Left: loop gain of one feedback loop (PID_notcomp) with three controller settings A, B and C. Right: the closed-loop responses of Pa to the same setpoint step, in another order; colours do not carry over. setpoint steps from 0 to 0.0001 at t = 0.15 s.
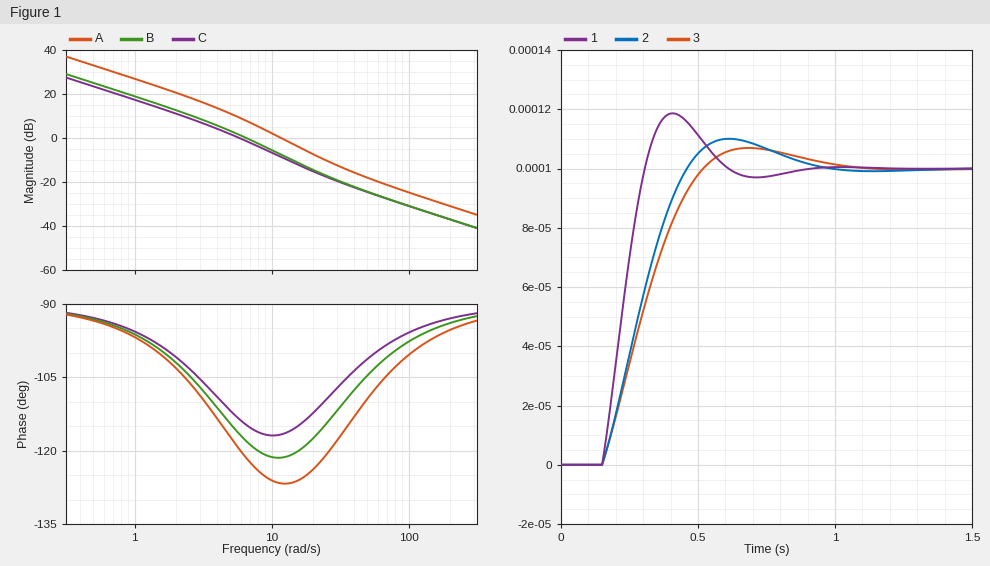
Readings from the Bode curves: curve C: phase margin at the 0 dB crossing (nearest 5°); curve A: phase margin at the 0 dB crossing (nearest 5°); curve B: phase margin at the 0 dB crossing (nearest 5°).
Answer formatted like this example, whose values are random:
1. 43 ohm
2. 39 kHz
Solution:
1. 65°
2. 55°
3. 60°
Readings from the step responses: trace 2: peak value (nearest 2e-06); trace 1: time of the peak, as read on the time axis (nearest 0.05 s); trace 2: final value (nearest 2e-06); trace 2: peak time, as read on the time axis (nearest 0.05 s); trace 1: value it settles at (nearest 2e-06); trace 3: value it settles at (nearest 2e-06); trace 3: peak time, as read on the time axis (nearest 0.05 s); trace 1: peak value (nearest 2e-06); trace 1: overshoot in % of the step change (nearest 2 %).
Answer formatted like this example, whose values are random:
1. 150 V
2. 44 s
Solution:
1. 0.000110
2. 0.40 s
3. 0.000100
4. 0.60 s
5. 0.000100
6. 0.000100
7. 0.70 s
8. 0.000118
9. 18 %
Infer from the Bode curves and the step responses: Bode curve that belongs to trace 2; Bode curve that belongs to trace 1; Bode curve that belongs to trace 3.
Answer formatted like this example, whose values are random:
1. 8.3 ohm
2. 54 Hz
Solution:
1. B
2. A
3. C
